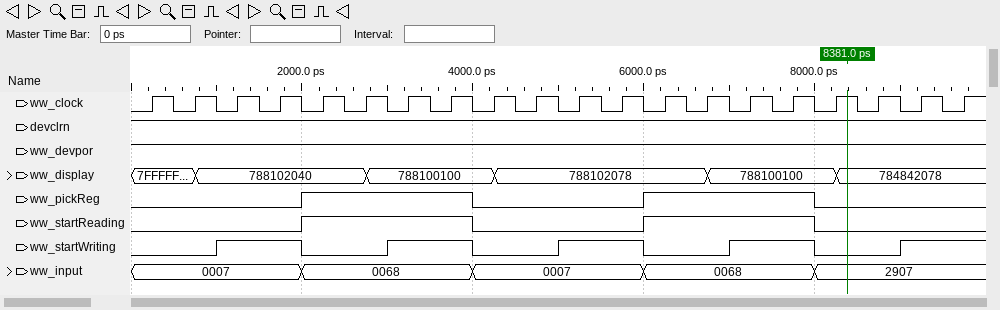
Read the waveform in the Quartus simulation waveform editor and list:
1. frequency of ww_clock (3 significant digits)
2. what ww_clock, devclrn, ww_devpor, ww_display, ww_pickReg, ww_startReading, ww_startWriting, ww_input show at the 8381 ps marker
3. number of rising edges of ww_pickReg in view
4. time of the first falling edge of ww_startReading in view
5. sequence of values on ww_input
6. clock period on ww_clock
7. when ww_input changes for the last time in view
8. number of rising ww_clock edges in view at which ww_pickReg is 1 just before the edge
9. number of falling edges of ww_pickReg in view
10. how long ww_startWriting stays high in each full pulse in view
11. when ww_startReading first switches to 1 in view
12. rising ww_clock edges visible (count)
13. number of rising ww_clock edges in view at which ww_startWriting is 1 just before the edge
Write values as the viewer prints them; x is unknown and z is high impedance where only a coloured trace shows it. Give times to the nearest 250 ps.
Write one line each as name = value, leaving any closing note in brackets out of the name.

frequency of ww_clock = 2.00 GHz
what ww_clock, devclrn, ww_devpor, ww_display, ww_pickReg, ww_startReading, ww_startWriting, ww_input show at the 8381 ps marker = ww_clock=1, devclrn=1, ww_devpor=1, ww_display=784842078, ww_pickReg=0, ww_startReading=0, ww_startWriting=0, ww_input=2907
number of rising edges of ww_pickReg in view = 2
time of the first falling edge of ww_startReading in view = 4000 ps
sequence of values on ww_input = 0007, 0068, 0007, 0068, 2907
clock period on ww_clock = 500 ps
when ww_input changes for the last time in view = 8000 ps
number of rising ww_clock edges in view at which ww_pickReg is 1 just before the edge = 8
number of falling edges of ww_pickReg in view = 2
how long ww_startWriting stays high in each full pulse in view = 1000 ps, 1000 ps, 1000 ps, 1000 ps
when ww_startReading first switches to 1 in view = 2000 ps
rising ww_clock edges visible = 20
number of rising ww_clock edges in view at which ww_startWriting is 1 just before the edge = 10
